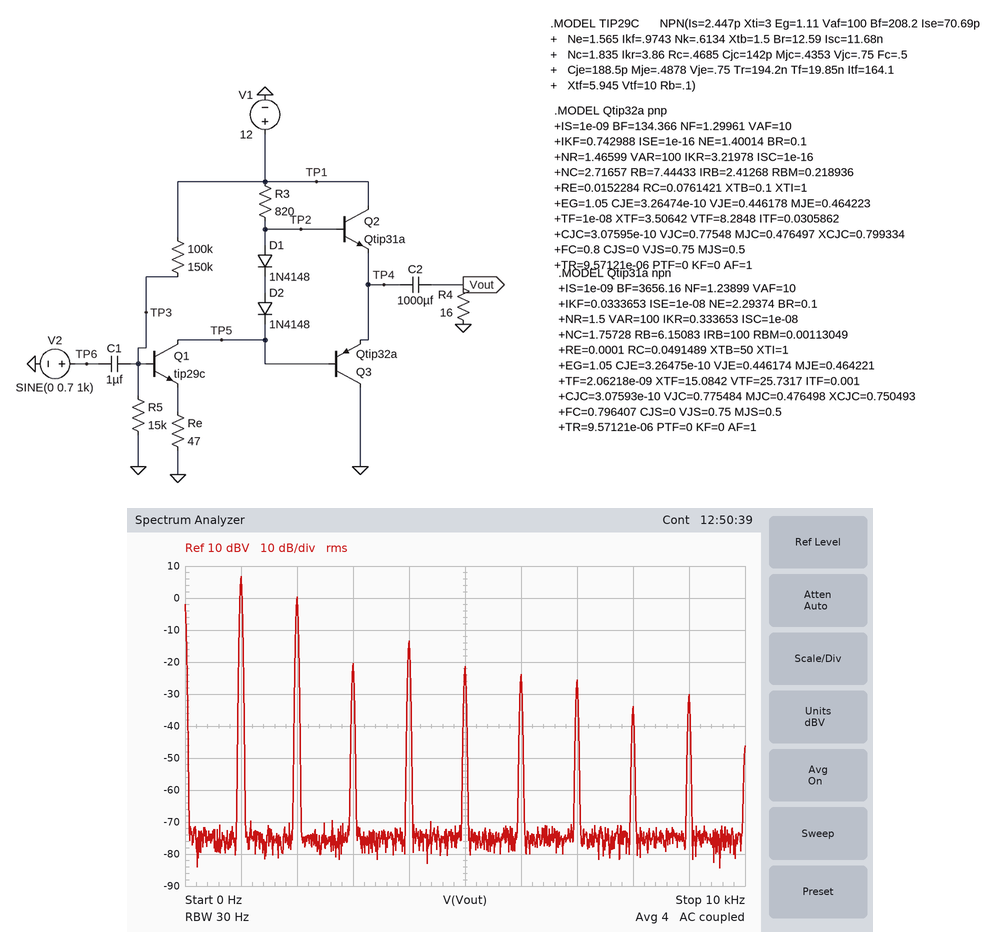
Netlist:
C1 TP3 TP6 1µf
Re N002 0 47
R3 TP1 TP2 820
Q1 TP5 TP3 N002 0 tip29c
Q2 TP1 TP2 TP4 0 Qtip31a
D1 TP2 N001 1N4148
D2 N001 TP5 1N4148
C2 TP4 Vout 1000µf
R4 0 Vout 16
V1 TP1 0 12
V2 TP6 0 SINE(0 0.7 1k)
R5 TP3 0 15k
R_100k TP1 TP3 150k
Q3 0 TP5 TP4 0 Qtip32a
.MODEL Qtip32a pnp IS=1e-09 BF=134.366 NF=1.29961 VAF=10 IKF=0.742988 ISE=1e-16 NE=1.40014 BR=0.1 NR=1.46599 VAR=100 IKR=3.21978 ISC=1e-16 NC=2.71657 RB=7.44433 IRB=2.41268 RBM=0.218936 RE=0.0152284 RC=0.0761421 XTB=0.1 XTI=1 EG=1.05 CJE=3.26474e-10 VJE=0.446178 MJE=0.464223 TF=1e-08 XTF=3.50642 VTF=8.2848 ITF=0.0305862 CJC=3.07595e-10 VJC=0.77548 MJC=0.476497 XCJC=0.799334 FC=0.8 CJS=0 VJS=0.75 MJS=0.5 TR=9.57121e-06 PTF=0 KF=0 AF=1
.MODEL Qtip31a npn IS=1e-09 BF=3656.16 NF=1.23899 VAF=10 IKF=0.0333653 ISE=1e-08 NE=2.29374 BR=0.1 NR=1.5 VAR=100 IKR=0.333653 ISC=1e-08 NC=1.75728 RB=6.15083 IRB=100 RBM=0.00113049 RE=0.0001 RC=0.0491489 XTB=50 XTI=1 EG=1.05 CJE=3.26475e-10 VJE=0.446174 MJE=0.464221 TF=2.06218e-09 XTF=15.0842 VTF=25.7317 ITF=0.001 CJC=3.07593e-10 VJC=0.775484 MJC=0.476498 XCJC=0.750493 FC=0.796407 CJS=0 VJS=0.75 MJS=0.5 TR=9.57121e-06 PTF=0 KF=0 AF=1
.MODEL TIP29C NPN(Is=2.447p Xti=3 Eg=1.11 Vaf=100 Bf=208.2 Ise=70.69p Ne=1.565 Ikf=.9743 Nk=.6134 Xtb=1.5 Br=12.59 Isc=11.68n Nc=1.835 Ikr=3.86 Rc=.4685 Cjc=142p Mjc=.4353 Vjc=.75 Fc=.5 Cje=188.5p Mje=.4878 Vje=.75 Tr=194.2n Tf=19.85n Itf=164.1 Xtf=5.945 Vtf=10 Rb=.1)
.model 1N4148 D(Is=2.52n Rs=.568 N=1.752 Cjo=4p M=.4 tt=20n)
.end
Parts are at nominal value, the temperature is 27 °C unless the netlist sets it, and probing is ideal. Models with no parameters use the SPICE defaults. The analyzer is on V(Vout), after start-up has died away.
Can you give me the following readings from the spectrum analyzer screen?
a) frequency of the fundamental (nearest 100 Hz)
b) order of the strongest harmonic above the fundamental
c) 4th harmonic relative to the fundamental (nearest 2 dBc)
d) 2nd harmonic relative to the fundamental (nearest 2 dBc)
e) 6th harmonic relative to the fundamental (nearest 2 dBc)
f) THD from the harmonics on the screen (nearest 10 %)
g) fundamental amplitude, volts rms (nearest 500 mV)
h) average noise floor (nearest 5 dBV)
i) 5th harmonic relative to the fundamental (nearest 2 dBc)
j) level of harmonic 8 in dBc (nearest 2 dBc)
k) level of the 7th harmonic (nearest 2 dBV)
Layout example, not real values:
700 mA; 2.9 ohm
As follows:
1.0 kHz; 2; -20 dBc; -6 dBc; -30 dBc; 50 %; 2.0 V; -75 dBV; -28 dBc; -40 dBc; -26 dBV
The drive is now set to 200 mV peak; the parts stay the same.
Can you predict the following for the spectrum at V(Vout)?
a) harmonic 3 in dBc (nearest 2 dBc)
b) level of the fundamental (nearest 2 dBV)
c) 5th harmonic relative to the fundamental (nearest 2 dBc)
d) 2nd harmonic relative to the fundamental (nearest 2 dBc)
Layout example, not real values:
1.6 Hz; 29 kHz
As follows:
-24 dBc; 2 dBV; -38 dBc; -14 dBc
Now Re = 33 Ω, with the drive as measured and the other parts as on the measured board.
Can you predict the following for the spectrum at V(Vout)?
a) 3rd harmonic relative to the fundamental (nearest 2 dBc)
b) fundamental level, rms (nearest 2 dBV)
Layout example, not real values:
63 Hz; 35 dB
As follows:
-20 dBc; 8 dBV
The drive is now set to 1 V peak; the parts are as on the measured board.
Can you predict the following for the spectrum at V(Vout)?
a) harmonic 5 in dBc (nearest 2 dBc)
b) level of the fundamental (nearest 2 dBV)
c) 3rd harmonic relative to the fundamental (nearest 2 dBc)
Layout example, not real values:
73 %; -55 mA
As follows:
-24 dBc; 8 dBV; -22 dBc
